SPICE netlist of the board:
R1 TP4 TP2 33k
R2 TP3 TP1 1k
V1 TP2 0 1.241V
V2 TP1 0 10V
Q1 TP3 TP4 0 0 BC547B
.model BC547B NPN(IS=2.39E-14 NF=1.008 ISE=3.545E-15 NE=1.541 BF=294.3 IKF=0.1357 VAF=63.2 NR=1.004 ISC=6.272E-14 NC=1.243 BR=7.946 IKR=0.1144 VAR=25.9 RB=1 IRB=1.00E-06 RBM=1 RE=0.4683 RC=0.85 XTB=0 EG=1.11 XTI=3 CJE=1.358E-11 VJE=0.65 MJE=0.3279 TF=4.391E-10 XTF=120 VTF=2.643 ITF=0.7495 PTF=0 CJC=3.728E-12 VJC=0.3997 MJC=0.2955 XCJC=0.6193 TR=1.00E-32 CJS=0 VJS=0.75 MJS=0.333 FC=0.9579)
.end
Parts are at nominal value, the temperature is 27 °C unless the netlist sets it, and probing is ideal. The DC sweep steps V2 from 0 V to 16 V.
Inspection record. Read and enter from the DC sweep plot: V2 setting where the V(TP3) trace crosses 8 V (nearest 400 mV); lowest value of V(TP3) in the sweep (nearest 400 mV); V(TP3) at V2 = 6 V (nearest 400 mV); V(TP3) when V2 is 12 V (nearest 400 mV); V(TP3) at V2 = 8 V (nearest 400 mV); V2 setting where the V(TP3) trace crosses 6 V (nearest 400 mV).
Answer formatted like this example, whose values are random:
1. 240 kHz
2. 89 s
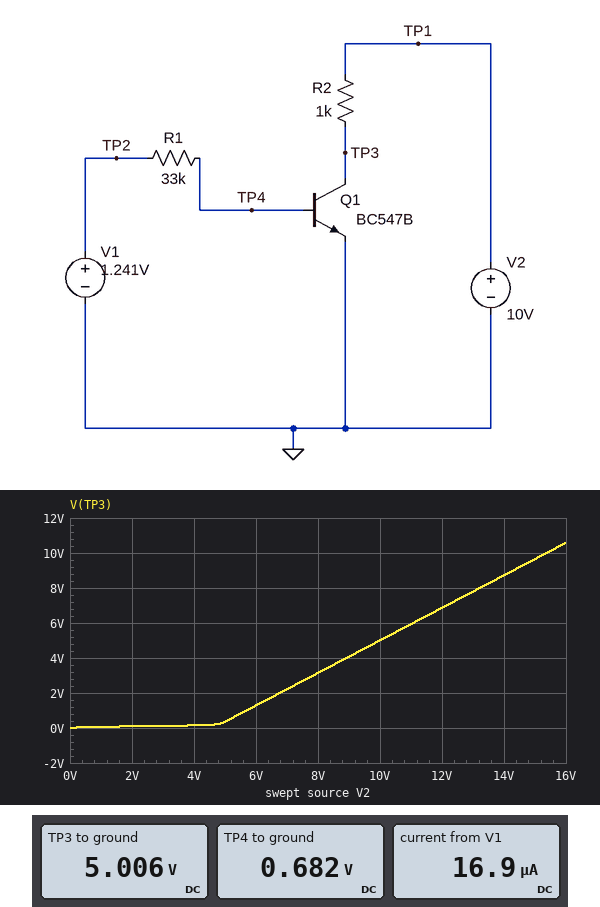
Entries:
1. 13.2 V
2. 0 V
3. 1.2 V
4. 6.8 V
5. 3.2 V
6. 11.2 V
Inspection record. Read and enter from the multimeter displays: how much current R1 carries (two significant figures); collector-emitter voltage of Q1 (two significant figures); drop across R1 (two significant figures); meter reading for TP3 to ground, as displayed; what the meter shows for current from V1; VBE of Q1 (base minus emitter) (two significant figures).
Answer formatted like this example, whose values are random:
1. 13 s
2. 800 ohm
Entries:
1. 17 µA
2. 5.0 V
3. 560 mV
4. 5.006 V
5. 16.9 µA
6. 680 mV
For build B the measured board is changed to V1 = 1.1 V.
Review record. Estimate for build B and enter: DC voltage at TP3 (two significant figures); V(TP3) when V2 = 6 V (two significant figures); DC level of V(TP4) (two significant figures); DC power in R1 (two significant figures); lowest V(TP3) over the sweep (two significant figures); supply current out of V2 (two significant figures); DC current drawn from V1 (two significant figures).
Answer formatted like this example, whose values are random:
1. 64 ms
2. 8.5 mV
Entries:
1. 6.1 V
2. 2.3 V
3. 670 mV
4. 5.5 µW
5. 5.1 mV
6. 3.9 mA
7. 13 µA
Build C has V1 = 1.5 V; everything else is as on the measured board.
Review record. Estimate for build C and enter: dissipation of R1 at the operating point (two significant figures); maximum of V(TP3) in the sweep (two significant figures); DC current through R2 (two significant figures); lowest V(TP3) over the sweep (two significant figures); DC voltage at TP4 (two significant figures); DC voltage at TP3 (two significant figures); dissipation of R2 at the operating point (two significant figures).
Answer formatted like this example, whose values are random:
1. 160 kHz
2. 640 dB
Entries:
1. 20 µW
2. 8.5 V
3. 6.9 mA
4. 5.6 mV
5. 690 mV
6. 3.1 V
7. 48 mW
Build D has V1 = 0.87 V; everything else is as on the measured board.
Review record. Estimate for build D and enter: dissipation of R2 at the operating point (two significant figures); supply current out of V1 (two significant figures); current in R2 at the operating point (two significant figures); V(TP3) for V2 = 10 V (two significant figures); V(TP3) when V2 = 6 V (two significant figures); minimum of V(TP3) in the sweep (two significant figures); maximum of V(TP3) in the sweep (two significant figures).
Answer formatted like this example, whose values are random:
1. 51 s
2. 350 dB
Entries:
1. 4.2 mW
2. 6.5 µA
3. 2.0 mA
4. 8.0 V
5. 4.1 V
6. 4.4 mV
7. 14 V
